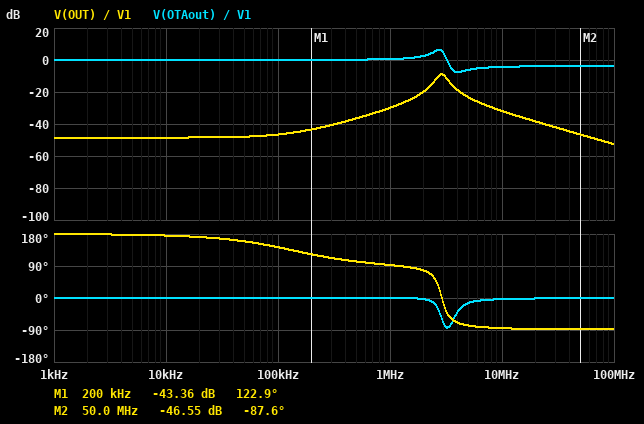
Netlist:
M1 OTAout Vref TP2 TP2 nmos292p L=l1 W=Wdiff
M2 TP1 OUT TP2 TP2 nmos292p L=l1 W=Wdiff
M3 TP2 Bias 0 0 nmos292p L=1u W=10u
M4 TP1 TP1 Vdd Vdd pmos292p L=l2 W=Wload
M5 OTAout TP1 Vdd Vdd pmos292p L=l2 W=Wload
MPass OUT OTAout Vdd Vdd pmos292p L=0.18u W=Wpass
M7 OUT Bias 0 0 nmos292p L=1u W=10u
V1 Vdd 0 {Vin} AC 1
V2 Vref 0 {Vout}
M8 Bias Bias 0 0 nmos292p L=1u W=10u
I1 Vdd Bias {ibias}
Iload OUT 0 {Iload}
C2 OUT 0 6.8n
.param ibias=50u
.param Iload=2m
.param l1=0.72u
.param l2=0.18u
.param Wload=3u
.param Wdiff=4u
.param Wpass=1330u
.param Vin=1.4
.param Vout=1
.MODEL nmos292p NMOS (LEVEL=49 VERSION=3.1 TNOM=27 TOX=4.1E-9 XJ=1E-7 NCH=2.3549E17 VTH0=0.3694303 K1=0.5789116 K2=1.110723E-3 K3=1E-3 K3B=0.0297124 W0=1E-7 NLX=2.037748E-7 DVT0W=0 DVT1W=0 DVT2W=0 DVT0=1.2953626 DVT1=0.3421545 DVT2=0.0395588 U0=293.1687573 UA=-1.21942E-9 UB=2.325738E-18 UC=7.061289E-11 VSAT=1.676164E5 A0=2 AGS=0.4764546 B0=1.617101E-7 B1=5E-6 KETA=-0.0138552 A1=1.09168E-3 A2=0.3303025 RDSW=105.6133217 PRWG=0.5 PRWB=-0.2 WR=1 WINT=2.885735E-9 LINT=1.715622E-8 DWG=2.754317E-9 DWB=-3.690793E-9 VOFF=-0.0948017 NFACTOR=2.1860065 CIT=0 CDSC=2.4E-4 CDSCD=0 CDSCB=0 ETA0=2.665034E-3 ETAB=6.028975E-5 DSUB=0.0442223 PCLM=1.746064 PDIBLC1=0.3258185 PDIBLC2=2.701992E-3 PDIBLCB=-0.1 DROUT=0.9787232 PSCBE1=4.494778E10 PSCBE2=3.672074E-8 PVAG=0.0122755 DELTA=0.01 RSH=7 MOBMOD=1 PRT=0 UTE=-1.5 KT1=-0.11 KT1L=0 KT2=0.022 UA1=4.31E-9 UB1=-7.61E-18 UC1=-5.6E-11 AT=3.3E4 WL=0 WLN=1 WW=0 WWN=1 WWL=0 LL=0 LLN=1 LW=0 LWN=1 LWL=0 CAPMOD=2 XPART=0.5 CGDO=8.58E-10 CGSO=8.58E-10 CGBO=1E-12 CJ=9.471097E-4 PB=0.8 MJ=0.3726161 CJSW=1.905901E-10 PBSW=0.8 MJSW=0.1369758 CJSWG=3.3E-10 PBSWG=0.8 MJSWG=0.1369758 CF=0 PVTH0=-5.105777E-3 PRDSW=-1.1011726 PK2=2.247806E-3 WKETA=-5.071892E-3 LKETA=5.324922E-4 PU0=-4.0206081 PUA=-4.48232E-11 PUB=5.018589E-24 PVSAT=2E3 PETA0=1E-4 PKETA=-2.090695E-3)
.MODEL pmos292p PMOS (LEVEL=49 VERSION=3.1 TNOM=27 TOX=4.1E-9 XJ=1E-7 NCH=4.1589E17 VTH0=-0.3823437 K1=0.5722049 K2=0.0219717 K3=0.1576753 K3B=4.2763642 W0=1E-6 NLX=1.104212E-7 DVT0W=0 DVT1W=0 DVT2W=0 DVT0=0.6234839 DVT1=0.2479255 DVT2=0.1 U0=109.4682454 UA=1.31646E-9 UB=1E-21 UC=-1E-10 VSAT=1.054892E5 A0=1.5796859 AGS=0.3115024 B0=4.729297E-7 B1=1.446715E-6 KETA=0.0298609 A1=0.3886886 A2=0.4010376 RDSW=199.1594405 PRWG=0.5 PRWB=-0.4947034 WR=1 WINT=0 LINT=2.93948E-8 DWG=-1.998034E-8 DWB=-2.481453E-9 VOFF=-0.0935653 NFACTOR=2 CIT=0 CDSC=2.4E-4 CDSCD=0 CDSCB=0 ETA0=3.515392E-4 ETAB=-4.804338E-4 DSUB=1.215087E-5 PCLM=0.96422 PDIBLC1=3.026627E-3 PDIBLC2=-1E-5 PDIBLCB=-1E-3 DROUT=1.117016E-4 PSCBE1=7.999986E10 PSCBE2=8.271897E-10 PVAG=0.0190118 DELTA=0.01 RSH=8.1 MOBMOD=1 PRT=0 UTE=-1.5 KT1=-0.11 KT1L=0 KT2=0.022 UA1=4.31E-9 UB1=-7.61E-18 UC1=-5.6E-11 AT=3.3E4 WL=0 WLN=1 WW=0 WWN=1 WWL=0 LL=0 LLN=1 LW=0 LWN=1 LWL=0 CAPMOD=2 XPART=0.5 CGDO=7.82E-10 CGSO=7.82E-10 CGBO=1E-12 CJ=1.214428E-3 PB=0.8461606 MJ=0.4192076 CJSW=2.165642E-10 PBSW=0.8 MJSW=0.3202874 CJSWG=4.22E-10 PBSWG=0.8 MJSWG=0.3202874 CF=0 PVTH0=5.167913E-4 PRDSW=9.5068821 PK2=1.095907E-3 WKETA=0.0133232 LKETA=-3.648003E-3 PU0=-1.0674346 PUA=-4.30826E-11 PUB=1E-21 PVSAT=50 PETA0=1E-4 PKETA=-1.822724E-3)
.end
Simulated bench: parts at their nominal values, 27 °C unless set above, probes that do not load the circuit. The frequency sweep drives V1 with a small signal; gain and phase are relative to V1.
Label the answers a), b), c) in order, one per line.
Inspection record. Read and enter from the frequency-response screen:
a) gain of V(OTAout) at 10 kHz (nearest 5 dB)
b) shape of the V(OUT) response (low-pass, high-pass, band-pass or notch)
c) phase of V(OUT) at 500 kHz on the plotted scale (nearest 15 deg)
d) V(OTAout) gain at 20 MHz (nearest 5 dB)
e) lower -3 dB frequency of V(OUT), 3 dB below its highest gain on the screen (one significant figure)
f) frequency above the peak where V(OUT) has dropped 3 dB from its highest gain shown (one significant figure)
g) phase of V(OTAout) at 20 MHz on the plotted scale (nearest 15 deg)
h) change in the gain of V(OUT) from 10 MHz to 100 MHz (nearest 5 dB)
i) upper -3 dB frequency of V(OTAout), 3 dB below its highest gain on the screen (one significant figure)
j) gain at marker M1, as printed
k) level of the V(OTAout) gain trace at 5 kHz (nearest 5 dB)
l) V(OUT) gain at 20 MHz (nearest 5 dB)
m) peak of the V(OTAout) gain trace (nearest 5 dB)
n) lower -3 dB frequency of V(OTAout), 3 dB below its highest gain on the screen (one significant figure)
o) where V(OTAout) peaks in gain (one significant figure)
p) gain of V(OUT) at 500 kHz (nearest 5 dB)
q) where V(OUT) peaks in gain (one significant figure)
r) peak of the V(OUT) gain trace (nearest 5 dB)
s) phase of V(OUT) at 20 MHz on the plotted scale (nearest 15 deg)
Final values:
a) 0 dB
b) band-pass
c) 105 deg
d) -5 dB
e) 3 MHz
f) 3 MHz
g) 0 deg
h) -20 dB
i) 3 MHz
j) -43.36 dB
k) 0 dB
l) -40 dB
m) 5 dB
n) 2 MHz
o) 3 MHz
p) -35 dB
q) 3 MHz
r) -10 dB
s) -90 deg
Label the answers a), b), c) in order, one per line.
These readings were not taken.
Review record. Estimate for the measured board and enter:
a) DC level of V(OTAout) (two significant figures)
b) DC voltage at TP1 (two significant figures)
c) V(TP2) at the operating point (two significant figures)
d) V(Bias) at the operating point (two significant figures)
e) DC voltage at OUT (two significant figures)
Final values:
a) 840 mV
b) 750 mV
c) 380 mV
d) 620 mV
e) 1.0 V
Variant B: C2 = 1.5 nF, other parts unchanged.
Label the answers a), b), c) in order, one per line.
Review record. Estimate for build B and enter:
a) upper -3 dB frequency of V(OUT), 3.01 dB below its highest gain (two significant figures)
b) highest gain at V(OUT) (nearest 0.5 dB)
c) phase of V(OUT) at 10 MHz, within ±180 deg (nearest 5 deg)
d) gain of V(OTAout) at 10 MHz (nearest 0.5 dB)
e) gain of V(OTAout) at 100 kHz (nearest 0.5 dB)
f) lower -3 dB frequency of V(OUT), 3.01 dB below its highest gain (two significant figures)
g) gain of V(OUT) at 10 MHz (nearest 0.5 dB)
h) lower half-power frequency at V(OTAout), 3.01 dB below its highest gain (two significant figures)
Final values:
a) 6.9 MHz
b) -2.5 dB
c) -75 deg
d) -6.5 dB
e) 0 dB
f) 5.5 MHz
g) -15.5 dB
h) 4.6 MHz
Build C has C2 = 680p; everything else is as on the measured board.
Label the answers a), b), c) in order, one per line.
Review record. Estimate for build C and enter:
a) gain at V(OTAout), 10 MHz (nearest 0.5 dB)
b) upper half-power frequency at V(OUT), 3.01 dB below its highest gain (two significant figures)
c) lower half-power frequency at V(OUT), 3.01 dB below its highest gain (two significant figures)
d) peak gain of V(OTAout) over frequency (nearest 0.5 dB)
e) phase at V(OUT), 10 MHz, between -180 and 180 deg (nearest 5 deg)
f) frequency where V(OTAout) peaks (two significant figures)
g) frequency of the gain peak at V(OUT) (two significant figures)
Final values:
a) 1.0 dB
b) 11 MHz
c) 7.9 MHz
d) 5.0 dB
e) -30 deg
f) 8.6 MHz
g) 9.1 MHz
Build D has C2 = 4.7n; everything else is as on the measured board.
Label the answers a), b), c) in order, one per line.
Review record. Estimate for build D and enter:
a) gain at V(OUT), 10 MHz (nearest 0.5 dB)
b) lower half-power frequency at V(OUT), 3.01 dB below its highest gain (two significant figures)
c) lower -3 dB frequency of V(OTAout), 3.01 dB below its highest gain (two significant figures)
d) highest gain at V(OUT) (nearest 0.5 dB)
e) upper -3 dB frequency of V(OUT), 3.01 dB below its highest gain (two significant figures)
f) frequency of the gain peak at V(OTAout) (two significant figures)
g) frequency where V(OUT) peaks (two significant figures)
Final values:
a) -28.5 dB
b) 3.1 MHz
c) 2.7 MHz
d) -7.0 dB
e) 3.9 MHz
f) 3.3 MHz
g) 3.5 MHz
